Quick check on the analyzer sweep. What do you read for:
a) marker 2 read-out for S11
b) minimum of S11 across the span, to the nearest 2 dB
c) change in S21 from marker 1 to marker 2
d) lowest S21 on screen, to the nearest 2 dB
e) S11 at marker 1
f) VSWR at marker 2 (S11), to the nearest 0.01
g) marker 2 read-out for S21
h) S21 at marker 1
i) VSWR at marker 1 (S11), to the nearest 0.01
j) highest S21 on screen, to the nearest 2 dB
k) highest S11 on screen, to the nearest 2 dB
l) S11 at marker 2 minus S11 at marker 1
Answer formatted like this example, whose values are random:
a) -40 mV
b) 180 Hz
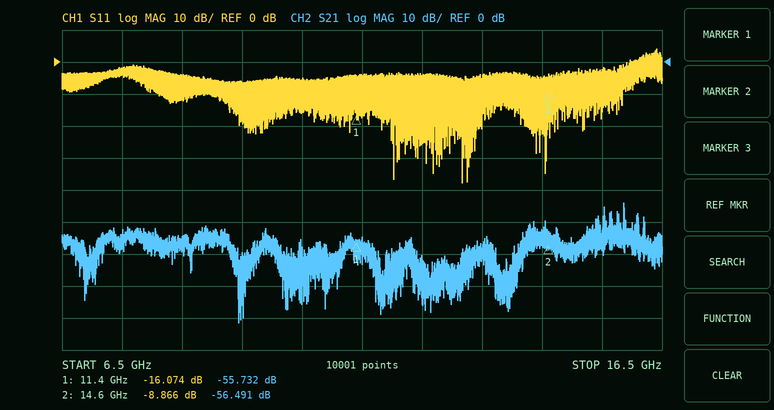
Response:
a) -8.866 dB
b) -38 dB
c) -0.759 dB
d) -82 dB
e) -16.074 dB
f) 2.13
g) -56.491 dB
h) -55.732 dB
i) 1.37
j) -44 dB
k) 4 dB
l) 7.208 dB
